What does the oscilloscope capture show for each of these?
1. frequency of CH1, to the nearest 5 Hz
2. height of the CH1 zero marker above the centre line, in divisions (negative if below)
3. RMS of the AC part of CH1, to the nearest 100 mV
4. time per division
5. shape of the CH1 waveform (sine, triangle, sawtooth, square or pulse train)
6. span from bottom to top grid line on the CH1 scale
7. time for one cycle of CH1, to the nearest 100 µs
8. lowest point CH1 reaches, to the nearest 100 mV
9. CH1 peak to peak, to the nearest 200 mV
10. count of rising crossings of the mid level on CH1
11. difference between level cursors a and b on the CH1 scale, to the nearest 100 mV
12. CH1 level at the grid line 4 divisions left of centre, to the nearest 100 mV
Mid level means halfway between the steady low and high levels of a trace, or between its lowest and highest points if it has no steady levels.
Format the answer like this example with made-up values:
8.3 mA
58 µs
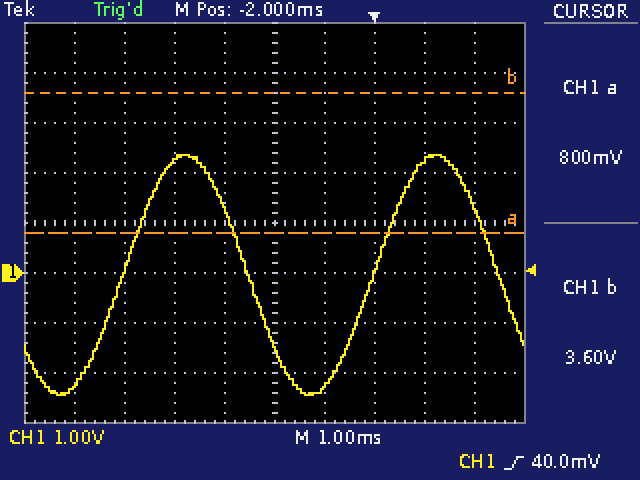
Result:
200 Hz
-1.0 div
1.7 V
1 ms
sine
8 V
5.0 ms
-2.4 V
4.8 V
2
2.8 V
-2.2 V
